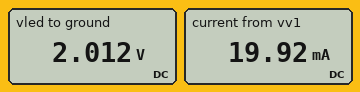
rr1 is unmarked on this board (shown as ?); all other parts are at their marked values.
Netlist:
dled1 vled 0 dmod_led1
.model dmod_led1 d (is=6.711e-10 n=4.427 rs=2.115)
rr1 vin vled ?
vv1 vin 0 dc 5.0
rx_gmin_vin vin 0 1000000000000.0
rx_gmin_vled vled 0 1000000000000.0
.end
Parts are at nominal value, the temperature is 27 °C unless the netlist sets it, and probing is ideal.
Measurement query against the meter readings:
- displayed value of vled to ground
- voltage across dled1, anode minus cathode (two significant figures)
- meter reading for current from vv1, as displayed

2.012 V
2.0 V
19.92 mA
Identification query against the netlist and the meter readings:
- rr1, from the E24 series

150 Ω
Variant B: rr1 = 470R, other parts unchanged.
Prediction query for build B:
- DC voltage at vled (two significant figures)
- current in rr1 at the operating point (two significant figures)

1.9 V
6.7 mA
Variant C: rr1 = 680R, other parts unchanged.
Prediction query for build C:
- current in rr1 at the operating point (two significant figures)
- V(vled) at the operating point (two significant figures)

4.7 mA
1.8 V
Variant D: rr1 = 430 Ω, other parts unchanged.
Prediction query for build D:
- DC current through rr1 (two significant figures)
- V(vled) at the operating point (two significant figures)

7.3 mA
1.9 V
